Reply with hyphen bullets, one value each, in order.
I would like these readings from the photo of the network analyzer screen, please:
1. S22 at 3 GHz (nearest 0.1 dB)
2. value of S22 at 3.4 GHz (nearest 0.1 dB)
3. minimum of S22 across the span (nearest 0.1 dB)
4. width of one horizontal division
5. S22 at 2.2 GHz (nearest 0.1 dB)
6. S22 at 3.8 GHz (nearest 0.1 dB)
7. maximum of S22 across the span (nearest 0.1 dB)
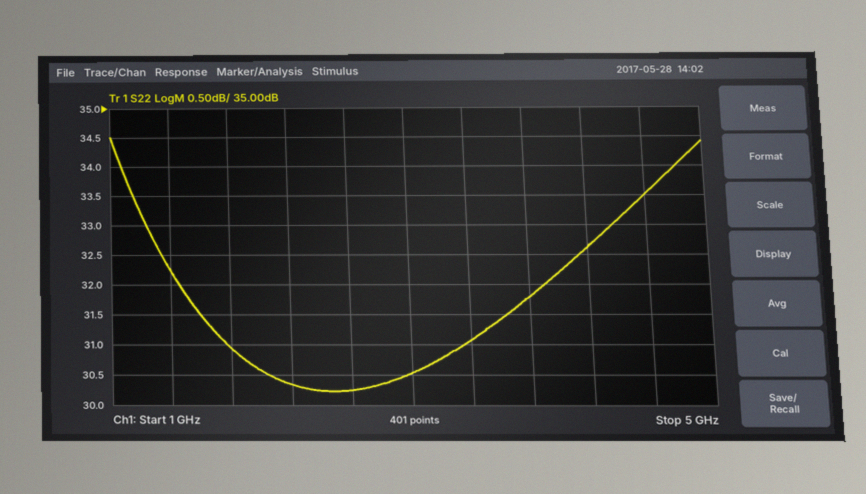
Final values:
- 30.5 dB
- 31.1 dB
- 30.2 dB
- 400 MHz
- 30.3 dB
- 31.8 dB
- 34.5 dB
